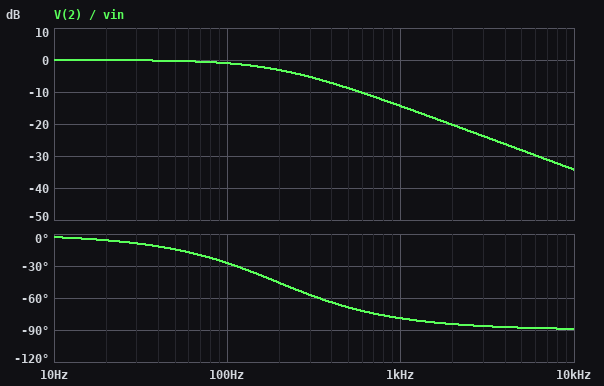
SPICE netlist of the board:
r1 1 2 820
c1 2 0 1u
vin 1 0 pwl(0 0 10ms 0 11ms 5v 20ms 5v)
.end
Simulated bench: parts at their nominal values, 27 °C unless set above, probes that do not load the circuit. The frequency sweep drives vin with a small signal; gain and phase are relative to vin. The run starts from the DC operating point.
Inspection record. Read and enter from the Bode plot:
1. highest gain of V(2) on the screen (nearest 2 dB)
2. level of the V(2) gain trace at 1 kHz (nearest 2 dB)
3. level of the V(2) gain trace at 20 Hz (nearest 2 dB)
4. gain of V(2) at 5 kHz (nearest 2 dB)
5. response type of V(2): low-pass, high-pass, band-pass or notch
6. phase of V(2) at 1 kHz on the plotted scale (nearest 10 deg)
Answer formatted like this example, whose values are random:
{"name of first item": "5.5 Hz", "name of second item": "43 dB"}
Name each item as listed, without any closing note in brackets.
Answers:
{"highest gain of V(2) on the screen": "0 dB", "level of the V(2) gain trace at 1 kHz": "-14 dB", "level of the V(2) gain trace at 20 Hz": "0 dB", "gain of V(2) at 5 kHz": "-28 dB", "response type of V(2): low-pass, high-pass, band-pass or notch": "low-pass", "phase of V(2) at 1 kHz on the plotted scale": "-80 deg"}
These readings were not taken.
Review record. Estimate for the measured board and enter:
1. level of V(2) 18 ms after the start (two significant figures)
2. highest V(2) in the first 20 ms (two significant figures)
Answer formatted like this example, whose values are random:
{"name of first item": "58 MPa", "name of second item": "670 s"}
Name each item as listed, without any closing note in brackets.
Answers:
{"level of V(2) 18 ms after the start": "5.0 V", "highest V(2) in the first 20 ms": "5.0 V"}
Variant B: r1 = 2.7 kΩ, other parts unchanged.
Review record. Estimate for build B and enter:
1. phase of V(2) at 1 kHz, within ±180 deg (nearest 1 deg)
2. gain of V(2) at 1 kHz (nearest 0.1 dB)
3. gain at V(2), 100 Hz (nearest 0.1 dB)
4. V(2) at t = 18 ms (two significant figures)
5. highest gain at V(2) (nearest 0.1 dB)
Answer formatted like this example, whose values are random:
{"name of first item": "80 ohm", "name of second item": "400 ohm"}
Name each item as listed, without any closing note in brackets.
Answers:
{"phase of V(2) at 1 kHz, within ±180 deg": "-87 deg", "gain of V(2) at 1 kHz": "-24.6 dB", "gain at V(2), 100 Hz": "-5.9 dB", "V(2) at t = 18 ms": "4.7 V", "highest gain at V(2)": "0 dB"}
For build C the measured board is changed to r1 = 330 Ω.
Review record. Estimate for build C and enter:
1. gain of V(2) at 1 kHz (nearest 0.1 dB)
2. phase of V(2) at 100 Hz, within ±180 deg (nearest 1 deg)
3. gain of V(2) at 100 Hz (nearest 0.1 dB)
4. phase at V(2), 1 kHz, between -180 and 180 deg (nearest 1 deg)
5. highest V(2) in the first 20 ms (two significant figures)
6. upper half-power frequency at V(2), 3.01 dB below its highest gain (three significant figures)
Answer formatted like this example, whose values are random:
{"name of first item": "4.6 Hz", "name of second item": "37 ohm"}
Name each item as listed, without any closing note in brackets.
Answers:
{"gain of V(2) at 1 kHz": "-7.2 dB", "phase of V(2) at 100 Hz, within ±180 deg": "-12 deg", "gain of V(2) at 100 Hz": "-0.2 dB", "phase at V(2), 1 kHz, between -180 and 180 deg": "-64 deg", "highest V(2) in the first 20 ms": "5.0 V", "upper half-power frequency at V(2), 3.01 dB below its highest gain": "482 Hz"}
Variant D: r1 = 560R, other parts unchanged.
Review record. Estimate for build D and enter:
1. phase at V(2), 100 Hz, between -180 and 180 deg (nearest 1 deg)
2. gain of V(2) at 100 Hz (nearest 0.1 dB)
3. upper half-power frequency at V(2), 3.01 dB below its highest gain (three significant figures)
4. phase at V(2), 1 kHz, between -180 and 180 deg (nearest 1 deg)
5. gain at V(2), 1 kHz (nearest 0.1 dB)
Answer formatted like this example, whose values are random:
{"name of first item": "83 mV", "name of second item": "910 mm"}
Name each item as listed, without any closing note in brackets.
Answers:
{"phase at V(2), 100 Hz, between -180 and 180 deg": "-19 deg", "gain of V(2) at 100 Hz": "-0.5 dB", "upper half-power frequency at V(2), 3.01 dB below its highest gain": "284 Hz", "phase at V(2), 1 kHz, between -180 and 180 deg": "-74 deg", "gain at V(2), 1 kHz": "-11.3 dB"}
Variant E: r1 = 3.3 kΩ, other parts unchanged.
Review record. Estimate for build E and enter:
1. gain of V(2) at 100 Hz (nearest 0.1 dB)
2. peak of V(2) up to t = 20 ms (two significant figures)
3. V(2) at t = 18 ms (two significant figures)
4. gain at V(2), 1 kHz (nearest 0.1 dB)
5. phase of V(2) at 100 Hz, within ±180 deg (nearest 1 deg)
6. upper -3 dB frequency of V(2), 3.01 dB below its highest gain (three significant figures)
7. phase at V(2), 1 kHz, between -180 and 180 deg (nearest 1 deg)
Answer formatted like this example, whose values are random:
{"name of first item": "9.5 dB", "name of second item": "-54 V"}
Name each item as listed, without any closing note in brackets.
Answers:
{"gain of V(2) at 100 Hz": "-7.2 dB", "peak of V(2) up to t = 20 ms": "4.7 V", "V(2) at t = 18 ms": "4.5 V", "gain at V(2), 1 kHz": "-26.3 dB", "phase of V(2) at 100 Hz, within ±180 deg": "-64 deg", "upper -3 dB frequency of V(2), 3.01 dB below its highest gain": "48.2 Hz", "phase at V(2), 1 kHz, between -180 and 180 deg": "-87 deg"}
